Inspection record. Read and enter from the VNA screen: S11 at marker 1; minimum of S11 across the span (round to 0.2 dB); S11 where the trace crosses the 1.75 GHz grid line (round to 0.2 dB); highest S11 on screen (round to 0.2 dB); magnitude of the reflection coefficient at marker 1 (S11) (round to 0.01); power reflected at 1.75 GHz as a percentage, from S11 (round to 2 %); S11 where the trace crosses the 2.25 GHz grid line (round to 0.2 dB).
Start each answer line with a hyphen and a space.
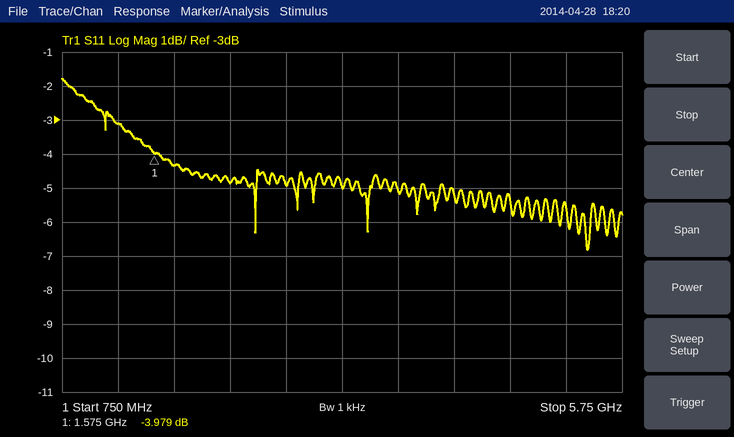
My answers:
- -3.979 dB
- -6.8 dB
- -4.4 dB
- -1.8 dB
- 0.63
- 36 %
- -4.8 dB
